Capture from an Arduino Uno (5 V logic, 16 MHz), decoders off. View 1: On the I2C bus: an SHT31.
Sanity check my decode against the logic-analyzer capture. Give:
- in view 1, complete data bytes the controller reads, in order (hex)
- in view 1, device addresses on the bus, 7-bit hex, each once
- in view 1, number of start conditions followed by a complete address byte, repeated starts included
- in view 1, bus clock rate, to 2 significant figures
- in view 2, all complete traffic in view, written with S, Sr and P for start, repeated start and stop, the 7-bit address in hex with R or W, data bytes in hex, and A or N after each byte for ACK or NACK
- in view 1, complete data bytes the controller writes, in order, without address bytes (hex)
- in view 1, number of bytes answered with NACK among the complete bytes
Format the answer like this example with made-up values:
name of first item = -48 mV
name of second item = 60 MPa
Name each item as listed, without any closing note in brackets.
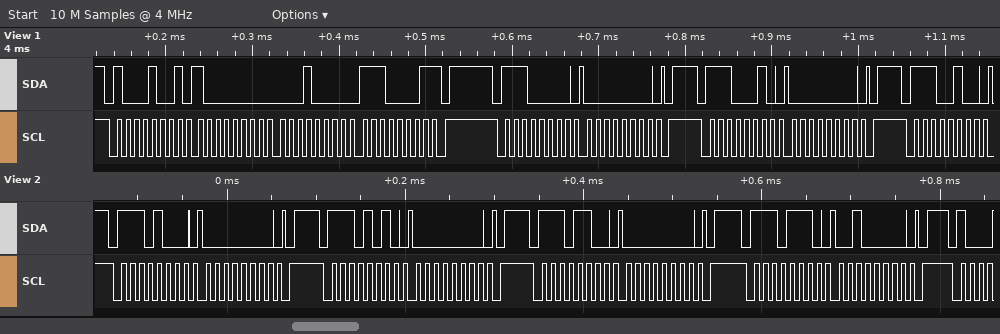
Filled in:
in view 1, complete data bytes the controller reads, in order = 80 10 E1
in view 1, device addresses on the bus, 7-bit hex, each once = 0x44 0x70 0x71 0x72
in view 1, number of start conditions followed by a complete address byte, repeated starts included = 4
in view 1, bus clock rate, to 2 significant figures = 100 kHz
in view 2, all complete traffic in view, written with S, Sr and P for start, repeated start and stop, the 7-bit address in hex with R or W, data bytes in hex, and A or N after each byte for ACK or NACK = S 74W A 00 A P S 75W A 00 A P S 76W A 00 A P S 77W A 20 A P
in view 1, complete data bytes the controller writes, in order, without address bytes = 00 00
in view 1, number of bytes answered with NACK among the complete bytes = 1
